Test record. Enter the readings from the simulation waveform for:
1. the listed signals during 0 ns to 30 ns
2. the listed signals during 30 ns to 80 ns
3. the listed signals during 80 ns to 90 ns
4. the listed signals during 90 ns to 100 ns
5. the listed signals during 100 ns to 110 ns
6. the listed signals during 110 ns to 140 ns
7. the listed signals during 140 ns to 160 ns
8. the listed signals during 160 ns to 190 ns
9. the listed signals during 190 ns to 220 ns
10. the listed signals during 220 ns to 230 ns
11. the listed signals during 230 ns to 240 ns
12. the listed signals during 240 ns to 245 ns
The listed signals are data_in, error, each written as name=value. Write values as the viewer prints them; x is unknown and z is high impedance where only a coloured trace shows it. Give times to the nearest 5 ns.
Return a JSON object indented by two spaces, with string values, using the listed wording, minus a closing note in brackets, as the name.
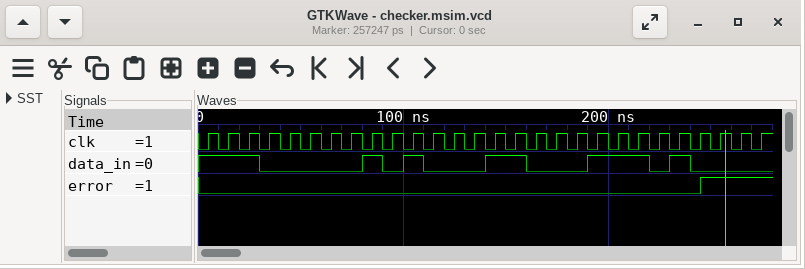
{
  "the listed signals during 0 ns to 30 ns": "data_in=1, error=0",
  "the listed signals during 30 ns to 80 ns": "data_in=0, error=0",
  "the listed signals during 80 ns to 90 ns": "data_in=1, error=0",
  "the listed signals during 90 ns to 100 ns": "data_in=0, error=0",
  "the listed signals during 100 ns to 110 ns": "data_in=1, error=0",
  "the listed signals during 110 ns to 140 ns": "data_in=0, error=0",
  "the listed signals during 140 ns to 160 ns": "data_in=1, error=0",
  "the listed signals during 160 ns to 190 ns": "data_in=0, error=0",
  "the listed signals during 190 ns to 220 ns": "data_in=1, error=0",
  "the listed signals during 220 ns to 230 ns": "data_in=0, error=0",
  "the listed signals during 230 ns to 240 ns": "data_in=1, error=0",
  "the listed signals during 240 ns to 245 ns": "data_in=0, error=0"
}
